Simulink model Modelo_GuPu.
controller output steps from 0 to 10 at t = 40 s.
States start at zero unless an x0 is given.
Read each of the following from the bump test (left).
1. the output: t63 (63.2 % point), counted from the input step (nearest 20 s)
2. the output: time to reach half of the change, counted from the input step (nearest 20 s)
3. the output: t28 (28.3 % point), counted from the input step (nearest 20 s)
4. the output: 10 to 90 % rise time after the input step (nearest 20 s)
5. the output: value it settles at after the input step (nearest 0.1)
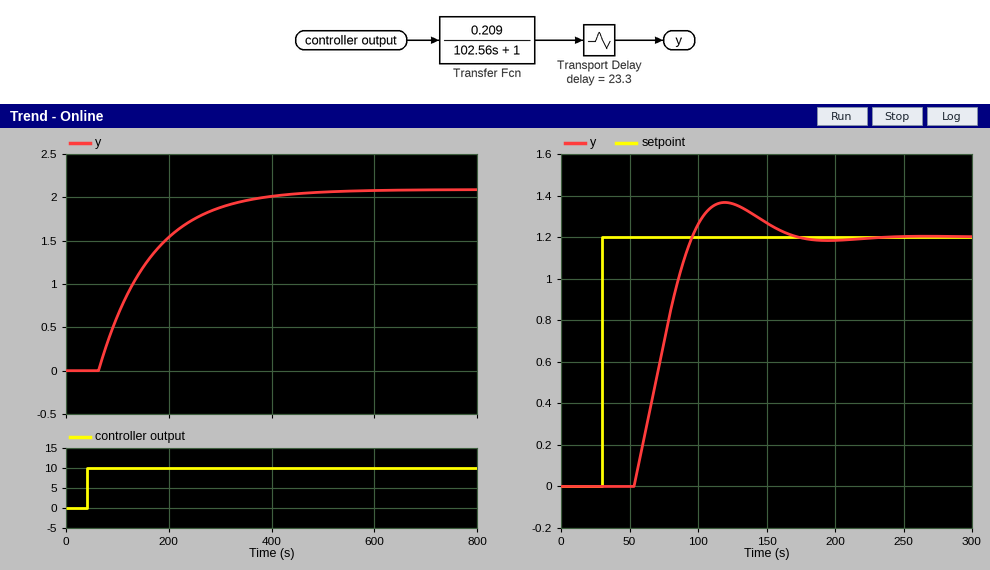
120 s
100 s
60 s
220 s
2.1
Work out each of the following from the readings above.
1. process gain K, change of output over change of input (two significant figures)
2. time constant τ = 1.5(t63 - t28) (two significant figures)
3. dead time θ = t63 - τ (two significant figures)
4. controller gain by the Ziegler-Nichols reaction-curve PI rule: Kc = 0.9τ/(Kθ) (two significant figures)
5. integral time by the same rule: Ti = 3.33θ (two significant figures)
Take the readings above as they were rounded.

0.21
90 s
30 s
13
100 s
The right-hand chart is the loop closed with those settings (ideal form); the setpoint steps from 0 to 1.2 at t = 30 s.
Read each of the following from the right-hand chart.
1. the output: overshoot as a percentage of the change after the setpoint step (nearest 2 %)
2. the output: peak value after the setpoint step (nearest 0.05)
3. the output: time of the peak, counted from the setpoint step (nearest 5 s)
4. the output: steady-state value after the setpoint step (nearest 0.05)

14 %
1.35
90 s
1.20
